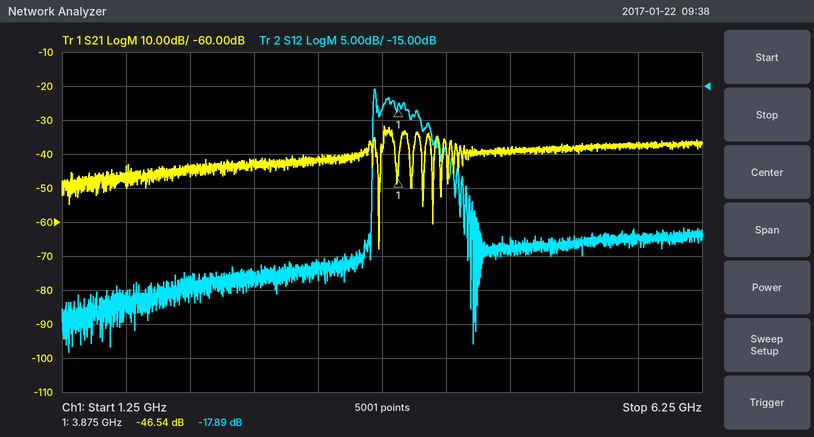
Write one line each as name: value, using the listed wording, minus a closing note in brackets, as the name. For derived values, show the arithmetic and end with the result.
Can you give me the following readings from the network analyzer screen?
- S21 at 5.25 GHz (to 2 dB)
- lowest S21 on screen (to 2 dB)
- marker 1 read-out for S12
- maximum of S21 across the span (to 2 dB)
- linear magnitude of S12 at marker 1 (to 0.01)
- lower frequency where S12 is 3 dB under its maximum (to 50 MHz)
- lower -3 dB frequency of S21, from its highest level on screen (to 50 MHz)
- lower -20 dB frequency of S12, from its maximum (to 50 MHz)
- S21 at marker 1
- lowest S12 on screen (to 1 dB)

S21 at 5.25 GHz: -38 dB
lowest S21 on screen: -68 dB
marker 1 read-out for S12: -17.89 dB
maximum of S21 across the span: -32 dB
linear magnitude of S12 at marker 1: 10^(-17.89/20) ≈ 0.13
lower frequency where S12 is 3 dB under its maximum: 3.70 GHz
lower -3 dB frequency of S21, from its highest level on screen: 3.75 GHz
lower -20 dB frequency of S12, from its maximum: 3.65 GHz
S21 at marker 1: -46.54 dB
lowest S12 on screen: -54 dB
